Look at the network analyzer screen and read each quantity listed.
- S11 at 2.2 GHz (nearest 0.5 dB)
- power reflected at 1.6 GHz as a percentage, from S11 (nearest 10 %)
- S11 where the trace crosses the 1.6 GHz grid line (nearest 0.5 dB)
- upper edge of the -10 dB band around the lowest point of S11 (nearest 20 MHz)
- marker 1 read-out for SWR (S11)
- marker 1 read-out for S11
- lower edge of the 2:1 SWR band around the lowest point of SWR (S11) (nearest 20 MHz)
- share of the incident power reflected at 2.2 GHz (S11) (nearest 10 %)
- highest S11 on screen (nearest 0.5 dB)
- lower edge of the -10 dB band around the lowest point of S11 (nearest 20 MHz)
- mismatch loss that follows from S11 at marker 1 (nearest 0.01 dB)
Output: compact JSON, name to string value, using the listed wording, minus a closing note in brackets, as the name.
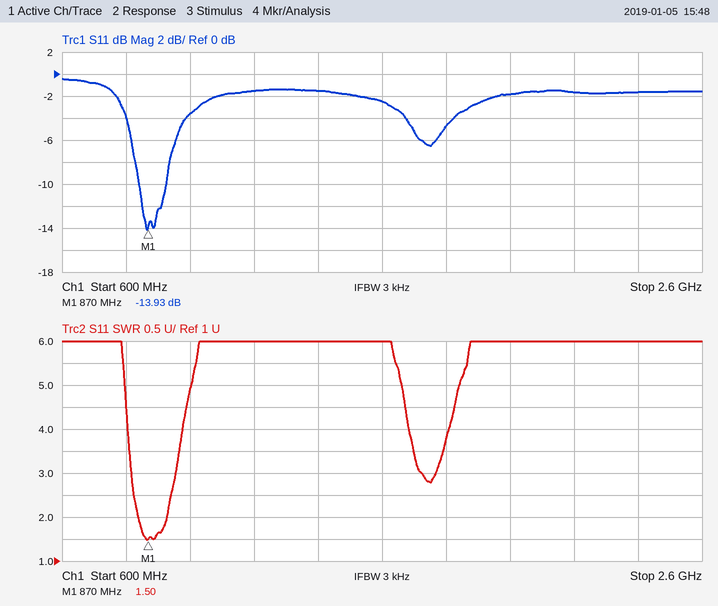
{"S11 at 2.2 GHz": "-1.5 dB", "power reflected at 1.6 GHz as a percentage, from S11": "60 %", "S11 where the trace crosses the 1.6 GHz grid line": "-2.5 dB", "upper edge of the -10 dB band around the lowest point of S11": "920 MHz", "marker 1 read-out for SWR": "1.50", "marker 1 read-out for S11": "-13.93 dB", "lower edge of the 2:1 SWR band around the lowest point of SWR (S11)": "840 MHz", "share of the incident power reflected at 2.2 GHz (S11)": "70 %", "highest S11 on screen": "-0.5 dB", "lower edge of the -10 dB band around the lowest point of S11": "840 MHz", "mismatch loss that follows from S11 at marker 1": "0.18 dB"}
